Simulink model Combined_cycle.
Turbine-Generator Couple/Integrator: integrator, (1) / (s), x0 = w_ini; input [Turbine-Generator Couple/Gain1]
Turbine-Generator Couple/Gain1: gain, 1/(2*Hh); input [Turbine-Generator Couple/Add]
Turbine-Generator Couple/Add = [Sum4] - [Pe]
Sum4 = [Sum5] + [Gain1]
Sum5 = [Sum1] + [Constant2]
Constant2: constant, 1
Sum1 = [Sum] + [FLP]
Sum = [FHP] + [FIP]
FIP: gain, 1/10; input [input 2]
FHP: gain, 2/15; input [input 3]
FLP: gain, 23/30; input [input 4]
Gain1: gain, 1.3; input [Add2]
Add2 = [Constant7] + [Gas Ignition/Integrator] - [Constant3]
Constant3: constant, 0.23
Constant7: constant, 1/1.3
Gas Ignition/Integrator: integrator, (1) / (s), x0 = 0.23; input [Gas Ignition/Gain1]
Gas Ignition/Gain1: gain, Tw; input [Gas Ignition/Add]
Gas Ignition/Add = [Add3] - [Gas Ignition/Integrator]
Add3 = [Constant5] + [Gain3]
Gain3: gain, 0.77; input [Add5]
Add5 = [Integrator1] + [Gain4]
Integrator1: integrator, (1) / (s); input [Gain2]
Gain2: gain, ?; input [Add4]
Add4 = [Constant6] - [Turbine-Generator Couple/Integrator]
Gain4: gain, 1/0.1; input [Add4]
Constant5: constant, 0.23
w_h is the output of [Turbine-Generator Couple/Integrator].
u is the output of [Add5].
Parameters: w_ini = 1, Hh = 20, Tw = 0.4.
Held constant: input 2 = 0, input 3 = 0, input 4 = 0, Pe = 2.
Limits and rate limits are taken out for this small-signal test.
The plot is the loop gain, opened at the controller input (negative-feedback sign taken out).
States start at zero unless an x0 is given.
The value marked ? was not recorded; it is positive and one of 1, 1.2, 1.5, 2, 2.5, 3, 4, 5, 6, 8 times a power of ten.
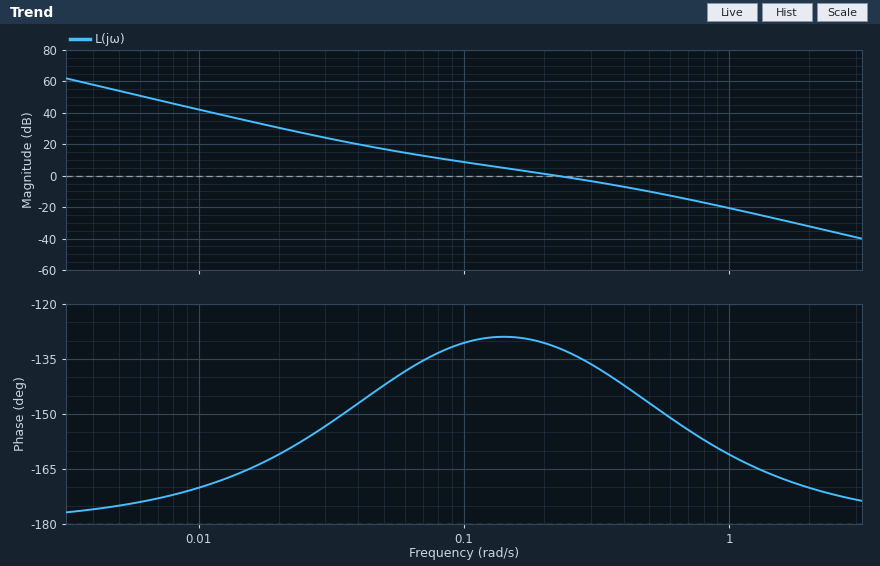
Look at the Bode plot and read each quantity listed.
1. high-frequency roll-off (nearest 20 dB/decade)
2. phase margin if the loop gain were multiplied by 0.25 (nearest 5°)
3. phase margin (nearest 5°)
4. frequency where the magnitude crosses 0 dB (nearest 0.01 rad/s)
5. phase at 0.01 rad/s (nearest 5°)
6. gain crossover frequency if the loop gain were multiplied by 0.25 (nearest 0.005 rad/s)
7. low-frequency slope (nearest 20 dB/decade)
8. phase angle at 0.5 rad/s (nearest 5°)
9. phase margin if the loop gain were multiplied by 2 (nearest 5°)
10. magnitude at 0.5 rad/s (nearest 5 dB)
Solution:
-40 dB/decade
45°
50°
0.22 rad/s
-170°
0.075 rad/s
-40 dB/decade
-145°
40°
-10 dB
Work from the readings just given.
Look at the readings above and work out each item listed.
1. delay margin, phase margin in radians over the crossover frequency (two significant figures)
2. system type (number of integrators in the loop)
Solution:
4.0 s
2
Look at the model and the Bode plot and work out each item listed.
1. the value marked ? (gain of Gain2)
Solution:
0.5
